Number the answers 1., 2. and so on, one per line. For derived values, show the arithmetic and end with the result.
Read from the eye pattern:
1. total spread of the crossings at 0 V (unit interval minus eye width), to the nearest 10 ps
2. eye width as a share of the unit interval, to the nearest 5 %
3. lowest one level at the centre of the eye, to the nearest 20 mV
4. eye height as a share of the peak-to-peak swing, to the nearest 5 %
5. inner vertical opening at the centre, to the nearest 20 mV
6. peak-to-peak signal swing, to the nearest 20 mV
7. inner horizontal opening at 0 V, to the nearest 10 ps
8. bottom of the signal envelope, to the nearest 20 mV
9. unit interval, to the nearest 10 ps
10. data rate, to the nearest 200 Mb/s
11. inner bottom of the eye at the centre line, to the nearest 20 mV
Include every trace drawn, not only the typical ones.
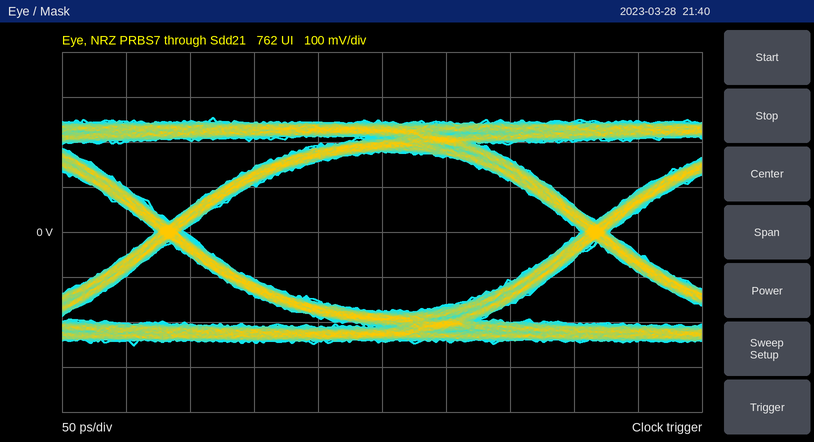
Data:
1. 20 ps
2. 310 ps / 330 ps ≈ 93.9 %, so 95 % to the nearest 5 %
3. 180 mV
4. 360 mV / 500 mV ≈ 72.0 %, so 70 % to the nearest 5 %
5. 360 mV
6. 500 mV
7. 310 ps
8. -260 mV
9. 330 ps
10. 3.0 Gb/s
11. -180 mV
